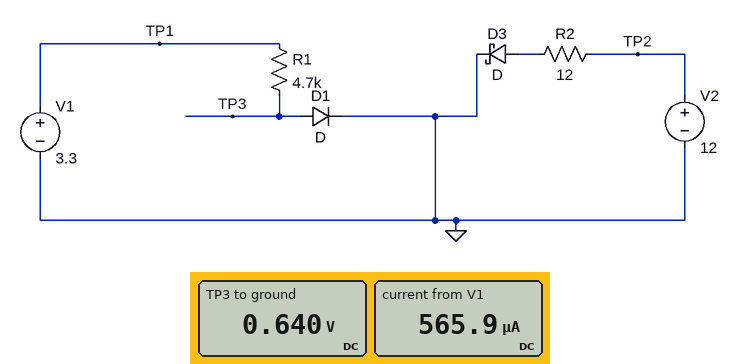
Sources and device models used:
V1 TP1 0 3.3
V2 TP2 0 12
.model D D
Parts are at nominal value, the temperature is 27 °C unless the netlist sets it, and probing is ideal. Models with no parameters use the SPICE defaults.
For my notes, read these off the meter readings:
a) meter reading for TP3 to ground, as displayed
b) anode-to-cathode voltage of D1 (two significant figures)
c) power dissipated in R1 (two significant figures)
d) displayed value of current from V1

0.640 V
640 mV
1.5 mW
565.9 µA
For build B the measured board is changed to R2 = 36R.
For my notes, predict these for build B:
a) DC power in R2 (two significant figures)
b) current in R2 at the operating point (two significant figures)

3.5 W
310 mA
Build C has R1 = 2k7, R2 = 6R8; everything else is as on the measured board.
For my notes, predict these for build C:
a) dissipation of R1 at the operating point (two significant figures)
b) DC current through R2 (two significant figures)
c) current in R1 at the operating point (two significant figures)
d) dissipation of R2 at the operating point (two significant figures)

2.6 mW
1.6 A
980 µA
18 W
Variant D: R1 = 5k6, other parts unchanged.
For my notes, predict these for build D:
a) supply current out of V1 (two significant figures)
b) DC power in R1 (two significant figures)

480 µA
1.3 mW
